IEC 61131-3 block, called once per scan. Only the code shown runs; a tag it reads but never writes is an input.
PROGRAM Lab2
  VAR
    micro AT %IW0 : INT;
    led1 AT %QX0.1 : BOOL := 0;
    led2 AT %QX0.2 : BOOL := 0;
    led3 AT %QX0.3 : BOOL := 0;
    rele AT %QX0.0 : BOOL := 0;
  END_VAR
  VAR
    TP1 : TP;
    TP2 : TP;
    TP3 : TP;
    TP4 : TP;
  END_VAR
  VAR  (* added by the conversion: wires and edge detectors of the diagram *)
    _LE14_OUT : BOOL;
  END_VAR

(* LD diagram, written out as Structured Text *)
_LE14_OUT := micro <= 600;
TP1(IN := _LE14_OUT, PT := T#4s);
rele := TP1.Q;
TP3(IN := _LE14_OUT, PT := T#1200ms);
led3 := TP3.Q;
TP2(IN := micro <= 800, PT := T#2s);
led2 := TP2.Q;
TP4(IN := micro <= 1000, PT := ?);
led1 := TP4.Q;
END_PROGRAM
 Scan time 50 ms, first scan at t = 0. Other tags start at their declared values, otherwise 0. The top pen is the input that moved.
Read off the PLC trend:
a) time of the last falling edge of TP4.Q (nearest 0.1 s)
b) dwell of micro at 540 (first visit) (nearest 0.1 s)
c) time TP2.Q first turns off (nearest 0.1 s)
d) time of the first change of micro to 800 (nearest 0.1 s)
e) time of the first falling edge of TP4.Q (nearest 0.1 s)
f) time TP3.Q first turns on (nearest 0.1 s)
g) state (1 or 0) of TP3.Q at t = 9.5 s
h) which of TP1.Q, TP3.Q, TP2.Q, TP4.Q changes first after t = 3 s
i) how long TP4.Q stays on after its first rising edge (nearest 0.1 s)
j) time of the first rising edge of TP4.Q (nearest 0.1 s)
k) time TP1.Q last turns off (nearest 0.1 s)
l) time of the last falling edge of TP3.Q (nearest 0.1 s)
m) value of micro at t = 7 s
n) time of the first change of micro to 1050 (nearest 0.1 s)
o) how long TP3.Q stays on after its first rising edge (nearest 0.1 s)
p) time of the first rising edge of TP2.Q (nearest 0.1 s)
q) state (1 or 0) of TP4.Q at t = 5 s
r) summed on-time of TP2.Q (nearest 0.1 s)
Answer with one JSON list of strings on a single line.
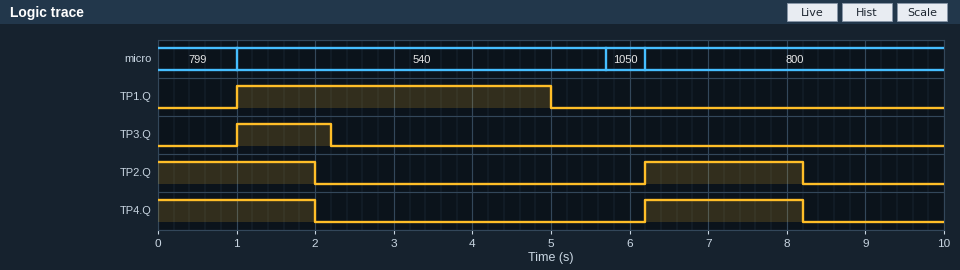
["8.2 s", "4.7 s", "2.0 s", "6.2 s", "2.0 s", "1.0 s", "0", "TP1.Q", "2.0 s", "6.2 s", "5.0 s", "2.2 s", "800", "5.7 s", "1.2 s", "6.2 s", "0", "4.0 s"]
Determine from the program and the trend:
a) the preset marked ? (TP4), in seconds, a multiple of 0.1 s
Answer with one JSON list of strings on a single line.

["2.0 s"]
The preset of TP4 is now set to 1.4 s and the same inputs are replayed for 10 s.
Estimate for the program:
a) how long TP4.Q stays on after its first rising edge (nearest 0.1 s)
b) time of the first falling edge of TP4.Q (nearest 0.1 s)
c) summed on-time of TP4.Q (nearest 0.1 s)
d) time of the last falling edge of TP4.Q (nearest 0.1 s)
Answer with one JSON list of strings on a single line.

["1.4 s", "1.4 s", "2.8 s", "7.6 s"]
